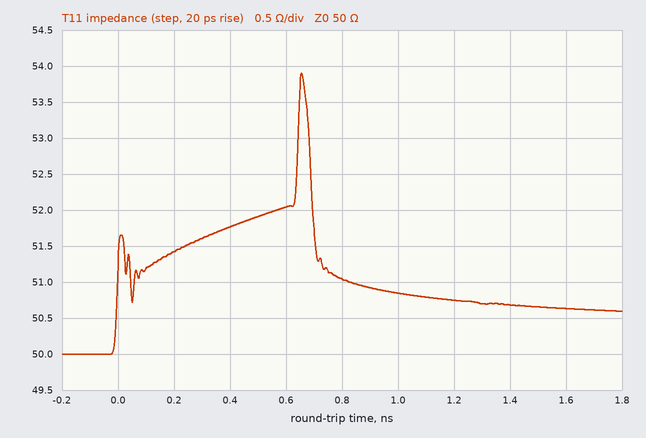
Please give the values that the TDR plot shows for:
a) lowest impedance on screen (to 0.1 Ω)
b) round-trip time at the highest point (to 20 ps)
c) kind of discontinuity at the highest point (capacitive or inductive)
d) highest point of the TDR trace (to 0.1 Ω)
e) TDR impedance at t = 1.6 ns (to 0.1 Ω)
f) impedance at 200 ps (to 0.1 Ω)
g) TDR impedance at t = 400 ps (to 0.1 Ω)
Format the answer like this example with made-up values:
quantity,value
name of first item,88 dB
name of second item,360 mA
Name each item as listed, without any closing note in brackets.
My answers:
quantity,value
lowest impedance on screen,50.0 Ω
round-trip time at the highest point,660 ps
kind of discontinuity at the highest point,inductive
highest point of the TDR trace,53.9 Ω
TDR impedance at t = 1.6 ns,50.6 Ω
impedance at 200 ps,51.4 Ω
TDR impedance at t = 400 ps,51.8 Ω
